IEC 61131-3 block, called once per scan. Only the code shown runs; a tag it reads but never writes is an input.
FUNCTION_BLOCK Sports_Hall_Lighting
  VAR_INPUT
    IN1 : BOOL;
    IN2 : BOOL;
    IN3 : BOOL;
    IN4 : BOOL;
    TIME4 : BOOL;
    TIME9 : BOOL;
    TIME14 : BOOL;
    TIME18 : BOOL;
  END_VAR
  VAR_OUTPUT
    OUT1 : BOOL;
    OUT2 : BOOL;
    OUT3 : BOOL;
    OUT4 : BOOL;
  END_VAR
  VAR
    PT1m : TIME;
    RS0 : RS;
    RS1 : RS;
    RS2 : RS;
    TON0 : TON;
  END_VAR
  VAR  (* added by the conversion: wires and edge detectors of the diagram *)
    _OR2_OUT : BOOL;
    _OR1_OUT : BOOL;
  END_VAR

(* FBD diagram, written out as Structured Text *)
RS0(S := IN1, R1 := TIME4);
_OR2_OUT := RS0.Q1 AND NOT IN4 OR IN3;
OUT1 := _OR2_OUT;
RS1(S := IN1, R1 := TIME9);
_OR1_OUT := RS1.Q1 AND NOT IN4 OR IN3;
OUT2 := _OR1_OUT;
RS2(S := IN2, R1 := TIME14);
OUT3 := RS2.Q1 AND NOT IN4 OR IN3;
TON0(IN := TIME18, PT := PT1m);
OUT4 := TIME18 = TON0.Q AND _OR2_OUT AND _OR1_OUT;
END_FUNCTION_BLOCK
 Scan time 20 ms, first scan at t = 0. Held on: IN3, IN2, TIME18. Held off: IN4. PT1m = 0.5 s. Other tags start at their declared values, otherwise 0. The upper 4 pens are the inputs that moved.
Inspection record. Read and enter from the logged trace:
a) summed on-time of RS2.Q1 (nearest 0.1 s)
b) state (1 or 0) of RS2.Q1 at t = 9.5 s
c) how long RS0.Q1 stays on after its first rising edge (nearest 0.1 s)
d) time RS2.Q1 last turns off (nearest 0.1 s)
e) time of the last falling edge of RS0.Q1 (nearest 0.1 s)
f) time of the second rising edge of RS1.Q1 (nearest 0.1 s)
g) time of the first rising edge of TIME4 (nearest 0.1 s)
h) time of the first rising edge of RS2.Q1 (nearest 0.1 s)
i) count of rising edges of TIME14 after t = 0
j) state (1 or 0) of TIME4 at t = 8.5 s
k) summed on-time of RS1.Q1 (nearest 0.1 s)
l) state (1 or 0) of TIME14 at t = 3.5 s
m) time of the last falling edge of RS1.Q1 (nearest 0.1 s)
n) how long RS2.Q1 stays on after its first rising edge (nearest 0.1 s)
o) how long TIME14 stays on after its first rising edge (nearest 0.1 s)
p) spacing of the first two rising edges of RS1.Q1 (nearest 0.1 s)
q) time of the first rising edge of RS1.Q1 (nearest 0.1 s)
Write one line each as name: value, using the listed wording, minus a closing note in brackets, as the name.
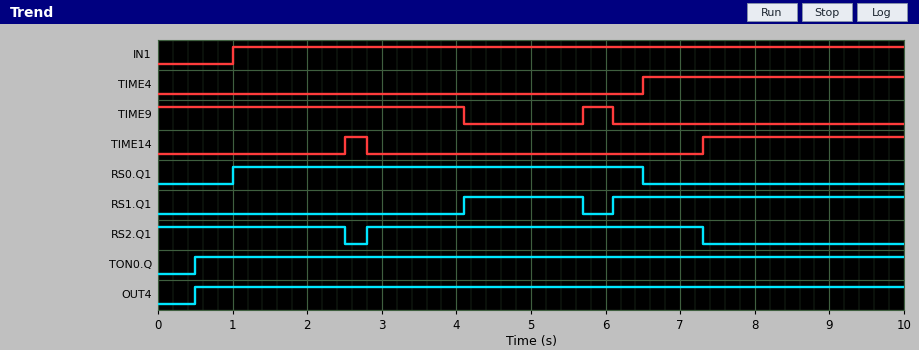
summed on-time of RS2.Q1: 7.0 s
state (1 or 0) of RS2.Q1 at t = 9.5 s: 0
how long RS0.Q1 stays on after its first rising edge: 5.5 s
time RS2.Q1 last turns off: 7.3 s
time of the last falling edge of RS0.Q1: 6.5 s
time of the second rising edge of RS1.Q1: 6.1 s
time of the first rising edge of TIME4: 6.5 s
time of the first rising edge of RS2.Q1: 2.8 s
count of rising edges of TIME14 after t = 0: 2
state (1 or 0) of TIME4 at t = 8.5 s: 1
summed on-time of RS1.Q1: 5.5 s
state (1 or 0) of TIME14 at t = 3.5 s: 0
time of the last falling edge of RS1.Q1: 5.7 s
how long RS2.Q1 stays on after its first rising edge: 4.5 s
how long TIME14 stays on after its first rising edge: 0.3 s
spacing of the first two rising edges of RS1.Q1: 2.0 s
time of the first rising edge of RS1.Q1: 4.1 s
